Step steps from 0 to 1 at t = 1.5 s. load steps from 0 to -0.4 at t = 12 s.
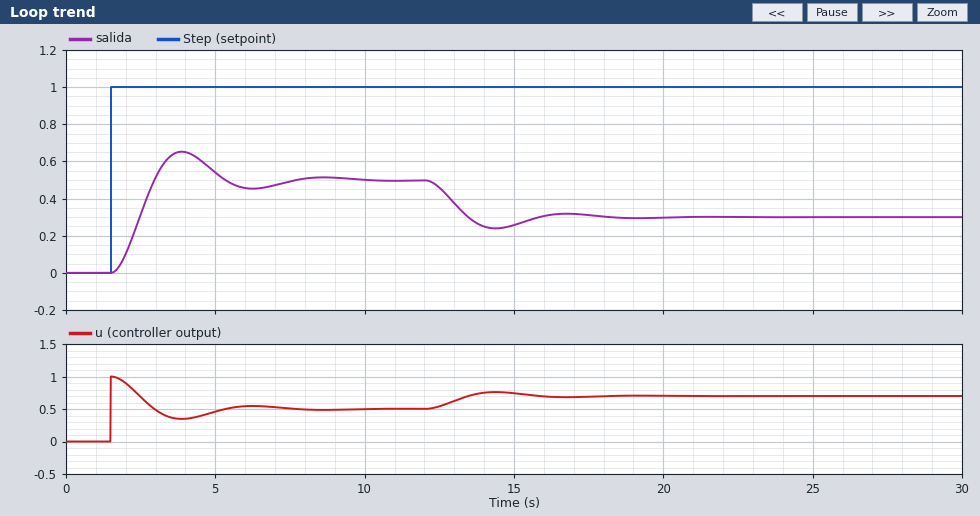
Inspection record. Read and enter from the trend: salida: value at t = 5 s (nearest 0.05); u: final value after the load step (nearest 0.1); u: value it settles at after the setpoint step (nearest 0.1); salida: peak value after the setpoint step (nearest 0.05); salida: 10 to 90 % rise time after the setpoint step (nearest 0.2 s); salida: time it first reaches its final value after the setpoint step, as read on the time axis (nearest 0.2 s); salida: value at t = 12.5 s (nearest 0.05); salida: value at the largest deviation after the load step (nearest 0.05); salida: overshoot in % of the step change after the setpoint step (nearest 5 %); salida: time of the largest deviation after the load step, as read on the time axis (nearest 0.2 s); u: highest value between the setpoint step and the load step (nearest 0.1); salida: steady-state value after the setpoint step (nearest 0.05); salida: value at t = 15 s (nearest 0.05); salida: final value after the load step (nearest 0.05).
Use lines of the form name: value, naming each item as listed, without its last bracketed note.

salida: value at t = 5 s: 0.55
u: final value after the load step: 0.7
u: value it settles at after the setpoint step: 0.5
salida: peak value after the setpoint step: 0.65
salida: 10 to 90 % rise time after the setpoint step: 1.0 s
salida: time it first reaches its final value after the setpoint step, as read on the time axis: 3.0 s
salida: value at t = 12.5 s: 0.45
salida: value at the largest deviation after the load step: 0.25
salida: overshoot in % of the step change after the setpoint step: 30 %
salida: time of the largest deviation after the load step, as read on the time axis: 14.4 s
u: highest value between the setpoint step and the load step: 1.0
salida: steady-state value after the setpoint step: 0.50
salida: value at t = 15 s: 0.25
salida: final value after the load step: 0.30
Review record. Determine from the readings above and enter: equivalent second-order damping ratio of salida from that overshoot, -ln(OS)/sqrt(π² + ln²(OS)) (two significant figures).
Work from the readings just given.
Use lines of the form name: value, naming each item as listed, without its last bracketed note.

equivalent second-order damping ratio of salida from that overshoot, -ln(OS)/sqrt(π² + ln²(OS)): 0.36
